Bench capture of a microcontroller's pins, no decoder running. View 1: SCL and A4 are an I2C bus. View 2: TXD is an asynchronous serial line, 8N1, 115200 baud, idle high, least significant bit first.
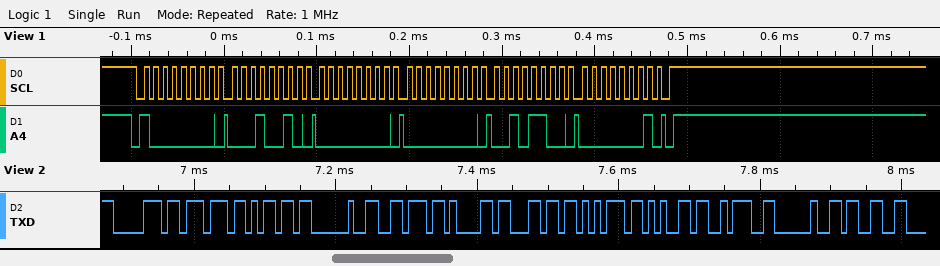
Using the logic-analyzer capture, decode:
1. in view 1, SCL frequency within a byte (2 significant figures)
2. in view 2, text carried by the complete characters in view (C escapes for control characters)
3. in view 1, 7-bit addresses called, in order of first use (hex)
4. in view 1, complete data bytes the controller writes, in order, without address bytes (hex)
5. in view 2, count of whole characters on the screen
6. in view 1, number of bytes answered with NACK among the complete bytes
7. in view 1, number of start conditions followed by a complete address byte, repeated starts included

100 kHz
"pwm value: 3"
0x40
12 00 00 2C 01
12
0
1
